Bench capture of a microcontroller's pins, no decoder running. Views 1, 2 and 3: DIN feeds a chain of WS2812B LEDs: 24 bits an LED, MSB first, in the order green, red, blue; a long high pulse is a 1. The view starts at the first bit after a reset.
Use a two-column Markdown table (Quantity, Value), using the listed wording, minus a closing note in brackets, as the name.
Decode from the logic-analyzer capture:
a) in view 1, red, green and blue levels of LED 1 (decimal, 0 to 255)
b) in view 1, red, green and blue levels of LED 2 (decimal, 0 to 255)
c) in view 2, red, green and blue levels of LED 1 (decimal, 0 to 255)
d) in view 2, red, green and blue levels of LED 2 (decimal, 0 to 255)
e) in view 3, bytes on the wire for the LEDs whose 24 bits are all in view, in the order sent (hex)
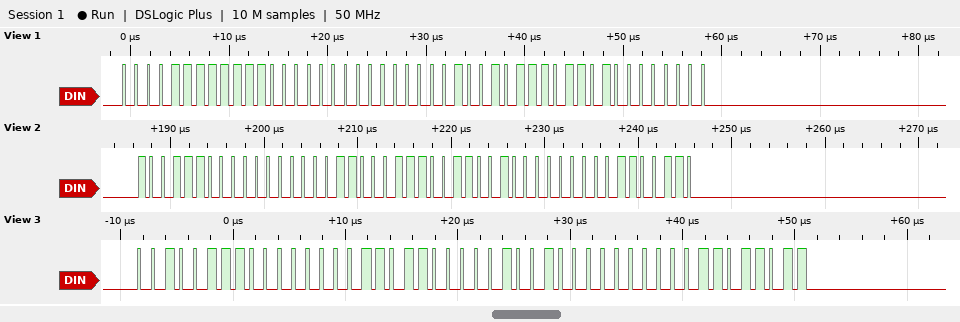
| Quantity | Value |
|---|---|
| in view 1, red, green and blue levels of LED 1 | 240, 15, 0 |
| in view 1, red, green and blue levels of LED 2 | 237, 18, 0 |
| in view 2, red, green and blue levels of LED 1 | 0, 156, 99 |
| in view 2, red, green and blue levels of LED 2 | 0, 153, 102 |
| in view 3, bytes on the wire for the LEDs whose 24 bits are all in view, in the order sent | 27 00 D8 24 00 DB |
